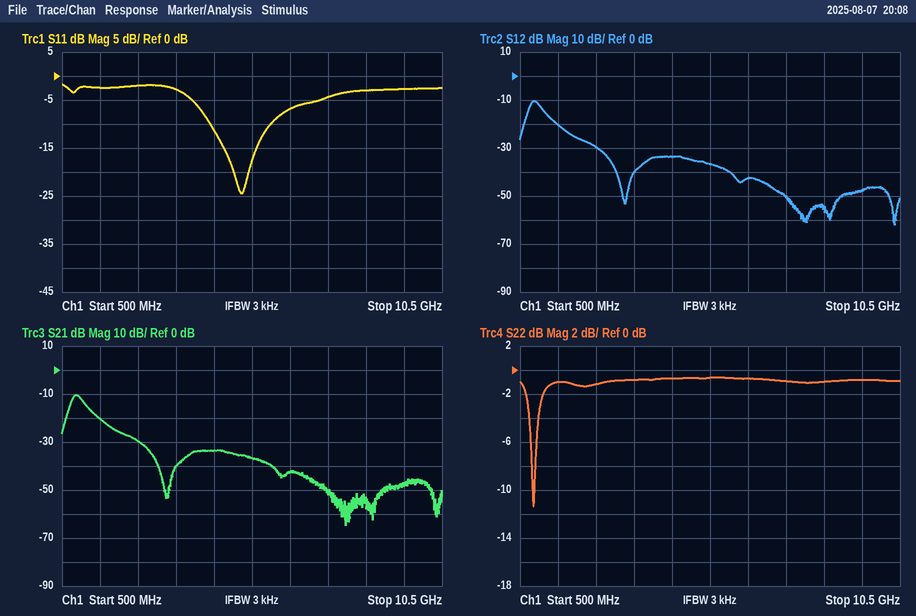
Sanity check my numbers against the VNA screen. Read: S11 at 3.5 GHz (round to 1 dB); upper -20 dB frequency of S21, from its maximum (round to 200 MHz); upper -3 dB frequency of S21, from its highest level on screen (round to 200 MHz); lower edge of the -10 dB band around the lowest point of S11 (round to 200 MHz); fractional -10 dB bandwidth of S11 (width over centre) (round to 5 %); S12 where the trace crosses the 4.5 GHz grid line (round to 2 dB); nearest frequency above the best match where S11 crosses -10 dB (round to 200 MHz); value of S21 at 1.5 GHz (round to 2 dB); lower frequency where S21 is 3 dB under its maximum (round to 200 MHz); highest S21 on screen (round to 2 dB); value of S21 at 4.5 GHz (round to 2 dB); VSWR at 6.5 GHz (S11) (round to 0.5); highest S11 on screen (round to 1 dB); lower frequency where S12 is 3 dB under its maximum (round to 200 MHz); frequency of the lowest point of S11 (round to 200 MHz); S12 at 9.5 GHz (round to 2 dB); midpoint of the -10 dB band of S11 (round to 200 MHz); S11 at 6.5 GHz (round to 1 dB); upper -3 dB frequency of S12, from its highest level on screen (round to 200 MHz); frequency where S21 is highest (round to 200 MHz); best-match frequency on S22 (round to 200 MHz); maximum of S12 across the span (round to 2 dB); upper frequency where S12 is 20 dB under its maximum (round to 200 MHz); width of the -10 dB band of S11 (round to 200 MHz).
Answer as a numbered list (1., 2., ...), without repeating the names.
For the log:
1. -3 dB
2. 2.6 GHz
3. 1.0 GHz
4. 4.4 GHz
5. 30 %
6. -34 dB
7. 6.0 GHz
8. -20 dB
9. 800 MHz
10. -10 dB
11. -34 dB
12. 2.5
13. -2 dB
14. 800 MHz
15. 5.2 GHz
16. -48 dB
17. 5.2 GHz
18. -7 dB
19. 1.0 GHz
20. 800 MHz
21. 800 MHz
22. -10 dB
23. 2.6 GHz
24. 1.6 GHz
